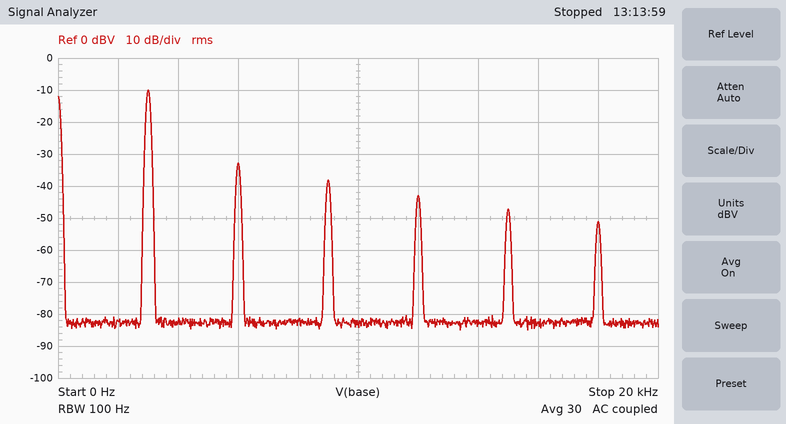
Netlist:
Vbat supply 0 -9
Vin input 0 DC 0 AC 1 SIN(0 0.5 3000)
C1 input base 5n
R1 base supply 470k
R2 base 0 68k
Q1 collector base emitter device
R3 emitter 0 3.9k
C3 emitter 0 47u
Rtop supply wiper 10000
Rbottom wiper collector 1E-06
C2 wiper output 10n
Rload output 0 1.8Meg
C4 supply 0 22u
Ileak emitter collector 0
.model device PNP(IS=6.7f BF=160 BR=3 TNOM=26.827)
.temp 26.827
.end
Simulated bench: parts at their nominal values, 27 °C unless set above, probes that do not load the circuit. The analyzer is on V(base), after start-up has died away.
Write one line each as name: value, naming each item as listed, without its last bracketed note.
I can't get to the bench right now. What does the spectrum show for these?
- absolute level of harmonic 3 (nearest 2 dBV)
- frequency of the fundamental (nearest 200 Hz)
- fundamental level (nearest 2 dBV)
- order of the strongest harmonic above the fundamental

absolute level of harmonic 3: -38 dBV
frequency of the fundamental: 3.0 kHz
fundamental level: -10 dBV
order of the strongest harmonic above the fundamental: 2
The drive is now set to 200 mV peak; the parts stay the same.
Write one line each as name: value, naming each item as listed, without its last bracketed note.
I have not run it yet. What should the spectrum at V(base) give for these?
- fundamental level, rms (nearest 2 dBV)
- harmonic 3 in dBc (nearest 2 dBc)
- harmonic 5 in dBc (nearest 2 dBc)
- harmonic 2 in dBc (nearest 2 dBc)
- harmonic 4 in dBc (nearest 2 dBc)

fundamental level, rms: -18 dBV
harmonic 3 in dBc: -34 dBc
harmonic 5 in dBc: -44 dBc
harmonic 2 in dBc: -26 dBc
harmonic 4 in dBc: -40 dBc
